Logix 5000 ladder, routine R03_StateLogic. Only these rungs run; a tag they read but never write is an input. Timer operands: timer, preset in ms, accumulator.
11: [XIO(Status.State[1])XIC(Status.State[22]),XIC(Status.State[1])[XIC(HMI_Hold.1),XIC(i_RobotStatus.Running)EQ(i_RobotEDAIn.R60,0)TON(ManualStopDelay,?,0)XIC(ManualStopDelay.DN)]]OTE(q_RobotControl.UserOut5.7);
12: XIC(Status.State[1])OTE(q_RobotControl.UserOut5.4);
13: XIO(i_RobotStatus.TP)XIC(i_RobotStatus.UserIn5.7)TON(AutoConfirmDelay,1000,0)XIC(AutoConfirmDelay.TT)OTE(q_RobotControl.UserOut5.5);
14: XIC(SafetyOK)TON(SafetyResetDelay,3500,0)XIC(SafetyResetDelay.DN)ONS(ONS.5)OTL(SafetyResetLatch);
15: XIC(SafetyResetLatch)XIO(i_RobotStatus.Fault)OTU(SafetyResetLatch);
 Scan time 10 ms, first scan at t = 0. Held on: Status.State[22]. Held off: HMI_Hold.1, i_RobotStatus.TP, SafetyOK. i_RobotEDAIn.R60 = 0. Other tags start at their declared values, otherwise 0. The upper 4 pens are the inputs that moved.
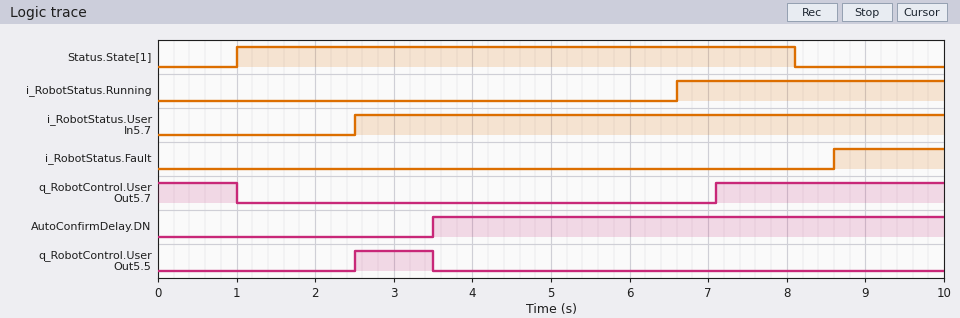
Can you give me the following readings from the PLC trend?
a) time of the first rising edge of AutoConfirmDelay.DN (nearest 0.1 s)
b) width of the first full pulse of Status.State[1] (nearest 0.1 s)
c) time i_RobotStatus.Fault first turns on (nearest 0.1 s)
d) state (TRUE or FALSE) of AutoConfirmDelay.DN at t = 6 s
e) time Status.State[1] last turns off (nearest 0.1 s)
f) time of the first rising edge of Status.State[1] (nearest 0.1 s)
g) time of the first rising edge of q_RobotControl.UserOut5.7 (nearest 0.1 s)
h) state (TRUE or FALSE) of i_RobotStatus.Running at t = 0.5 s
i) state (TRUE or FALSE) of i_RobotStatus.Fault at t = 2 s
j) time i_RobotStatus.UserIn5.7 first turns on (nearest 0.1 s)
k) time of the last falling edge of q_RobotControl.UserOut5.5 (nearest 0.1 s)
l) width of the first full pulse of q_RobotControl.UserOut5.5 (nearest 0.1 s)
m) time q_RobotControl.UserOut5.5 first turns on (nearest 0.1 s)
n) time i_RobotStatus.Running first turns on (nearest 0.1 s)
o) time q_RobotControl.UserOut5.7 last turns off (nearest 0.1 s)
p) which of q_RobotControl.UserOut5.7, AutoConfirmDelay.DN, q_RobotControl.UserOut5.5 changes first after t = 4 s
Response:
3.5 s
7.1 s
8.6 s
TRUE
8.1 s
1.0 s
7.1 s
FALSE
FALSE
2.5 s
3.5 s
1.0 s
2.5 s
6.6 s
1.0 s
q_RobotControl.UserOut5.7
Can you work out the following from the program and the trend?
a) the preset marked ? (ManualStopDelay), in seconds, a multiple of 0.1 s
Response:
0.5 s
